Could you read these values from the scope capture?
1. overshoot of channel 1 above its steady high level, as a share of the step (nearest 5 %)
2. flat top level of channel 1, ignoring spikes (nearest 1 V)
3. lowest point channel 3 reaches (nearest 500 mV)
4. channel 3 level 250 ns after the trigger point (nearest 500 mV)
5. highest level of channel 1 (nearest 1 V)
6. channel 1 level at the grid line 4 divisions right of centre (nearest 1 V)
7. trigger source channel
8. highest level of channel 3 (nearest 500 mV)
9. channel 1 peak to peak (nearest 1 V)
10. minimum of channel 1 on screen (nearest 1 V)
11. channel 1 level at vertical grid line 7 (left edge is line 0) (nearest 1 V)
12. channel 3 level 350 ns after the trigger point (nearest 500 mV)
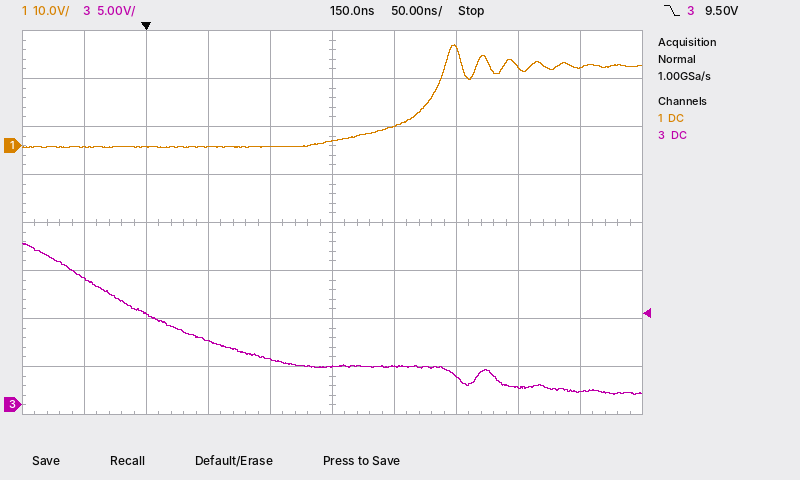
25 %
17 V
1.0 V
3.0 V
21 V
16 V
channel 3
17.0 V
21 V
0 V
20 V
1.5 V
